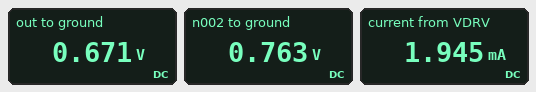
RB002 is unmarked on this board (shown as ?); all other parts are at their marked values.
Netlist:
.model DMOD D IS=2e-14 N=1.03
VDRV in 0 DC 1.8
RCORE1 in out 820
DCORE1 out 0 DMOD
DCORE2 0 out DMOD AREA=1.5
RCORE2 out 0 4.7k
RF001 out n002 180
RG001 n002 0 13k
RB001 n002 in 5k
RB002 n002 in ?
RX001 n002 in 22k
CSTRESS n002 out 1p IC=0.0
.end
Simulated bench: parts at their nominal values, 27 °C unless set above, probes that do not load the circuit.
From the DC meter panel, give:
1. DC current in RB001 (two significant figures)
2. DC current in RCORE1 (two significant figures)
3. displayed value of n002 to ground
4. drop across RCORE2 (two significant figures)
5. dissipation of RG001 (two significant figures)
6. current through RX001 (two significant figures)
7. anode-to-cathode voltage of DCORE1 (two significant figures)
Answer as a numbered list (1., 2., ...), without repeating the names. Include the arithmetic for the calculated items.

1. (1.8 V - 763 mV) / 5 kΩ = 210 µA
2. (1.8 V - 671 mV) / 820 Ω = 1.4 mA
3. 0.763 V
4. 671 mV = 670 mV
5. (763 mV)^2 / 13 kΩ = 45 µW
6. (1.8 V - 763 mV) / 22 kΩ = 47 µA
7. 671 mV = 670 mV
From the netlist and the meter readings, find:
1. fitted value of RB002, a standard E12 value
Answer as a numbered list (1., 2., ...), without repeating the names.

1. 3.3 kΩ
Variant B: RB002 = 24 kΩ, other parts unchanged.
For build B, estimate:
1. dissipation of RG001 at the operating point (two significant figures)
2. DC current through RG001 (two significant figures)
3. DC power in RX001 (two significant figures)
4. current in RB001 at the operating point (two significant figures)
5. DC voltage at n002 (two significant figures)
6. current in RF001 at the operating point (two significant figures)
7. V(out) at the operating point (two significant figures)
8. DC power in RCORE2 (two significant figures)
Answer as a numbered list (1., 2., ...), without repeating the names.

1. 39 µW
2. 55 µA
3. 54 µW
4. 220 µA
5. 710 mV
6. 260 µA
7. 670 mV
8. 95 µW
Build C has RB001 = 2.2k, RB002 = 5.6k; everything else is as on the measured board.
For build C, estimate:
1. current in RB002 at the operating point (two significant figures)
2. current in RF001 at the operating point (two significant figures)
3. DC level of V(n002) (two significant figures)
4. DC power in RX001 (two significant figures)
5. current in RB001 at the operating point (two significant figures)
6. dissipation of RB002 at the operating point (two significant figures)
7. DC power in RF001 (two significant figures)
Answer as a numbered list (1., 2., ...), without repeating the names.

1. 180 µA
2. 630 µA
3. 790 mV
4. 47 µW
5. 460 µA
6. 180 µW
7. 71 µW
